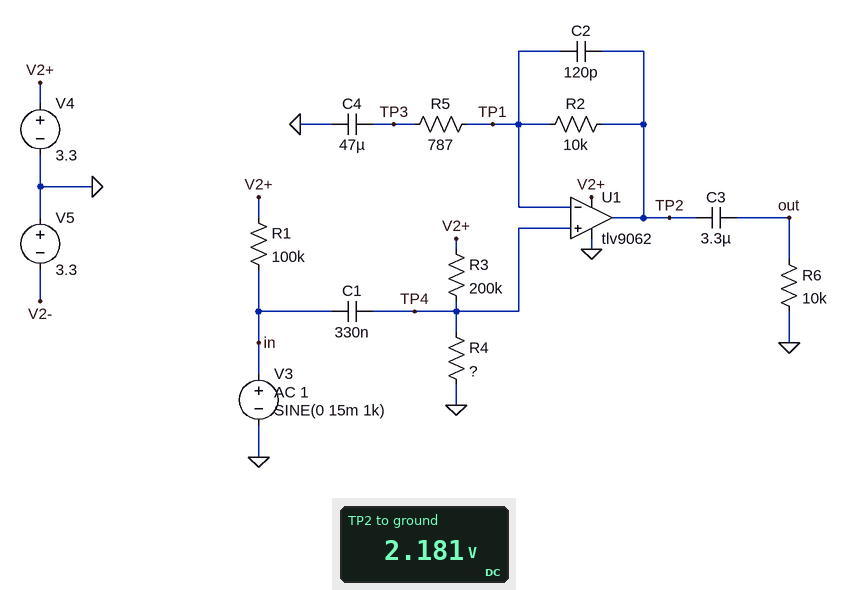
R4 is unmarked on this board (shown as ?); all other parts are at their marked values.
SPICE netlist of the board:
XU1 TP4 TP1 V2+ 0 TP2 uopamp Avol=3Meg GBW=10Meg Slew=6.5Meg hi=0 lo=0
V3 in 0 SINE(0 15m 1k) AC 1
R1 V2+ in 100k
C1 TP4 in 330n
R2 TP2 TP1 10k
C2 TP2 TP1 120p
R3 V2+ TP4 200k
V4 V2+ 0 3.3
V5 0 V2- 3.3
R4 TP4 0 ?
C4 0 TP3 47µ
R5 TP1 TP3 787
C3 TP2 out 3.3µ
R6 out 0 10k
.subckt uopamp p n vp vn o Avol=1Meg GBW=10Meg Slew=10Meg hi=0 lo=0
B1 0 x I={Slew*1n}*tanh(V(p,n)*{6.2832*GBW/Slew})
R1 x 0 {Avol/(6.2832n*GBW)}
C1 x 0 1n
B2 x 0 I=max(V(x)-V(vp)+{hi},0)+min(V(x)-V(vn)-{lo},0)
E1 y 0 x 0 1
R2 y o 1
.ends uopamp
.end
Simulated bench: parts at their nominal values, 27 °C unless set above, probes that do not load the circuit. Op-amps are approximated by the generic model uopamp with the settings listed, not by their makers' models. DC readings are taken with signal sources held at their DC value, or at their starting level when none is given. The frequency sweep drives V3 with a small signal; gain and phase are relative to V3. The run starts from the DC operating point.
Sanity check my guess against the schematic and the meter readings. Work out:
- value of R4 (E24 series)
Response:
390 kΩ
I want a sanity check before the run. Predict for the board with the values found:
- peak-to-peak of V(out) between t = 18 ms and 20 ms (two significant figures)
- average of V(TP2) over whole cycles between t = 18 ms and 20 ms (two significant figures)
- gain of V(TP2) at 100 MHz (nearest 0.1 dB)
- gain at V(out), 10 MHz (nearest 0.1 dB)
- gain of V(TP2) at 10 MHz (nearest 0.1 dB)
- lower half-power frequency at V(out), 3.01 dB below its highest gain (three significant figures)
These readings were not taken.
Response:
410 mV
2.2 V
-20.1 dB
-3.6 dB
-3.6 dB
8.37 Hz
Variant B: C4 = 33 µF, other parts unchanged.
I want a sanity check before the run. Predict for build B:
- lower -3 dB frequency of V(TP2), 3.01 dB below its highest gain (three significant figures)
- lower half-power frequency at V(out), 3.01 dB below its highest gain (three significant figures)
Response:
7.68 Hz
9.65 Hz
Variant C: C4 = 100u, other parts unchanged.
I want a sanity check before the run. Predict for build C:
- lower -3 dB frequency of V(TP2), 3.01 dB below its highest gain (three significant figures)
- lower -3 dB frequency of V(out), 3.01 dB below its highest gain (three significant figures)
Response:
4.48 Hz
7.09 Hz
